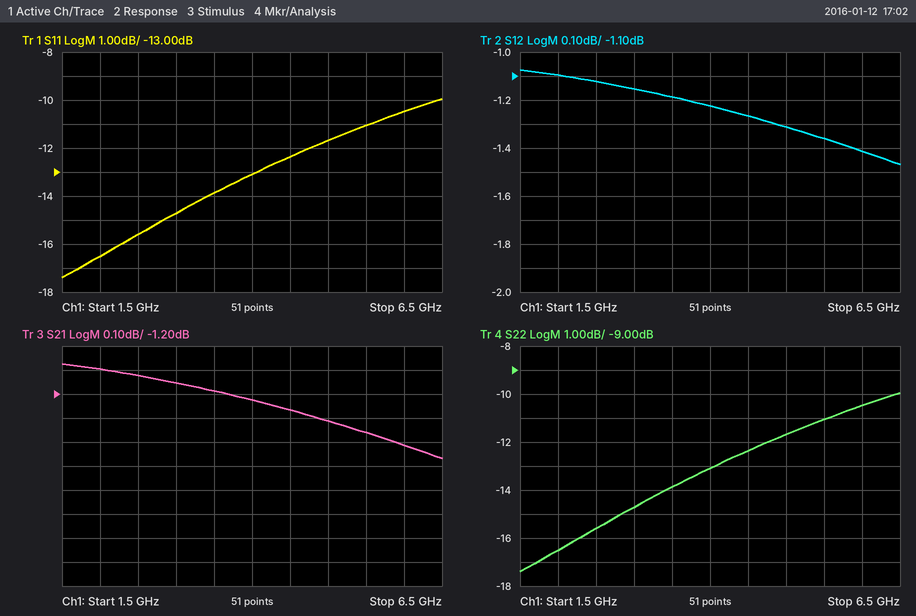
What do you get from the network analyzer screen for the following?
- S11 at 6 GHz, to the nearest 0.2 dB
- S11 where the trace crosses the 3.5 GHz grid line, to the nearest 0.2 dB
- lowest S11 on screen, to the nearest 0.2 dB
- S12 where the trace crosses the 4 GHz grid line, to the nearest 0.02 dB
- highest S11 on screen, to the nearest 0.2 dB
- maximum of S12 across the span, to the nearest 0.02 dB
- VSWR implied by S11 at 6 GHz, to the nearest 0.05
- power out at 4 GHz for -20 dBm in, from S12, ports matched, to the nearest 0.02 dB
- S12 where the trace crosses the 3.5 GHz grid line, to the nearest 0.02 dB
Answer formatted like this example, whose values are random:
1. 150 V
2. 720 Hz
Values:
1. -10.4 dB
2. -13.8 dB
3. -17.4 dB
4. -1.22 dB
5. -10.0 dB
6. -1.08 dB
7. 1.85
8. -21.22 dBm
9. -1.18 dB
